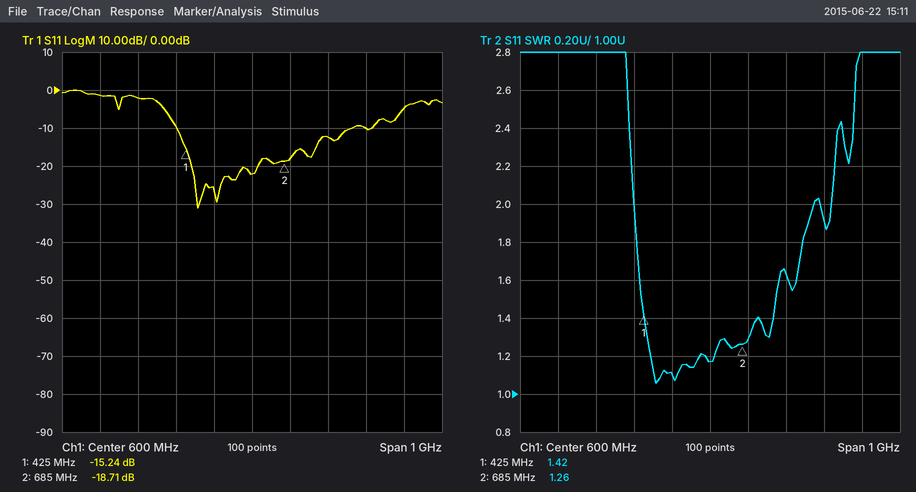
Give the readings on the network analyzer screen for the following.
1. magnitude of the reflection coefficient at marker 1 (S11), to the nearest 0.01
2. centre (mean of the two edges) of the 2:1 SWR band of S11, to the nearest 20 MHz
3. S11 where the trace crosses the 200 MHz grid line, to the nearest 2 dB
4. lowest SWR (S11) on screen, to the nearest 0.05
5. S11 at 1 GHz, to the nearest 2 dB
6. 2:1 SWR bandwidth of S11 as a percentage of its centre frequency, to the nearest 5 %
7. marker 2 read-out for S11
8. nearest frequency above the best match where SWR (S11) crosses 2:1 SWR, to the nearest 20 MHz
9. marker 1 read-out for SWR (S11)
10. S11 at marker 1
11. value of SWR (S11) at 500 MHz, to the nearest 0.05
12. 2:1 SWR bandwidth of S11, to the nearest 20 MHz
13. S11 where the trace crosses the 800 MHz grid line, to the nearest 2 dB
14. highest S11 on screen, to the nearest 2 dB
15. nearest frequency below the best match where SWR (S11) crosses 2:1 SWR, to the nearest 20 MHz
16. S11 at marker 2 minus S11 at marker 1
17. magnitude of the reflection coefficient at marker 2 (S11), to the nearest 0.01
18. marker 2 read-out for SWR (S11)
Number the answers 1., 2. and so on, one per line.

1. 0.17
2. 640 MHz
3. -2 dB
4. 1.05
5. -4 dB
6. 75 %
7. -18.71 dB
8. 880 MHz
9. 1.42
10. -15.24 dB
11. 1.10
12. 480 MHz
13. -12 dB
14. 0 dB
15. 400 MHz
16. -3.47 dB
17. 0.12
18. 1.26
